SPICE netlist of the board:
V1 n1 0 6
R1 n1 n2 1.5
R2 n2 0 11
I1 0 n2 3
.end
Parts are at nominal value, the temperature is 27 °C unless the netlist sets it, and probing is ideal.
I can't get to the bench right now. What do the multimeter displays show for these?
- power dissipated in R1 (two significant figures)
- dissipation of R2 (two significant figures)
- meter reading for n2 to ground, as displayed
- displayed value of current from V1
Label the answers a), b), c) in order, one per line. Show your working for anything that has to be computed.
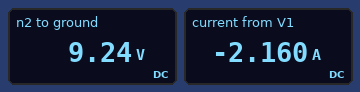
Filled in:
a) (9.24 V - 6 V)^2 / 1.5 Ω = 7.0 W
b) (9.24 V)^2 / 11 Ω = 7.8 W
c) 9.24 V
d) -2.160 A
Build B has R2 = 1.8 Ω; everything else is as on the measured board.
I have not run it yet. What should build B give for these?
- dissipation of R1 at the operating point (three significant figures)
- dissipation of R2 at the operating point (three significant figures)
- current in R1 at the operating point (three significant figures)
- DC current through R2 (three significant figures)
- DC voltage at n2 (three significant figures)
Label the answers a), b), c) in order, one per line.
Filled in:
a) 49.6 mW
b) 18.2 W
c) 182 mA
d) 3.18 A
e) 5.73 V
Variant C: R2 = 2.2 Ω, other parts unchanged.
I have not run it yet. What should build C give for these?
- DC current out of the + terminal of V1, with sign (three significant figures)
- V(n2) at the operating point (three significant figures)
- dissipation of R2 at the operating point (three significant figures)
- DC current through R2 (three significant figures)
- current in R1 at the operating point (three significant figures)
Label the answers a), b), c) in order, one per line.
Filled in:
a) -162 mA
b) 6.24 V
c) 17.7 W
d) 2.84 A
e) 162 mA
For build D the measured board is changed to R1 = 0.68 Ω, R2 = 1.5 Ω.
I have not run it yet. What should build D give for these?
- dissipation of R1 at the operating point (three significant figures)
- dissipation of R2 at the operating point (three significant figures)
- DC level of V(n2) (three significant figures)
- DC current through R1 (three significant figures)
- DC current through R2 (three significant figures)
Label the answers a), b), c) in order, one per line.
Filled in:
a) 322 mW
b) 20.4 W
c) 5.53 V
d) 688 mA
e) 3.69 A
